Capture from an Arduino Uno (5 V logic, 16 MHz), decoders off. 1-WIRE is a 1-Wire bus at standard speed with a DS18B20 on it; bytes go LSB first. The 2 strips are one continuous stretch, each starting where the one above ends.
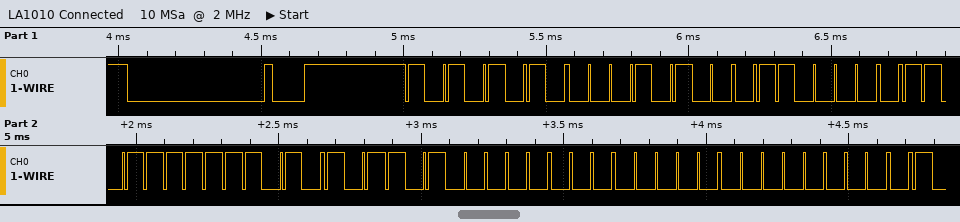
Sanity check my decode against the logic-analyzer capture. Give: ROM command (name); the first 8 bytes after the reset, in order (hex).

Match ROM
55 28 06 FB AB 05 00 00
